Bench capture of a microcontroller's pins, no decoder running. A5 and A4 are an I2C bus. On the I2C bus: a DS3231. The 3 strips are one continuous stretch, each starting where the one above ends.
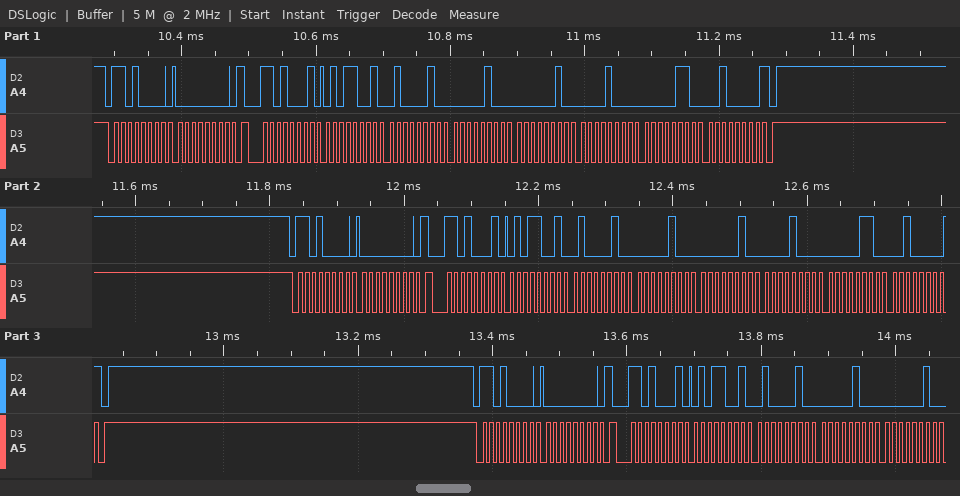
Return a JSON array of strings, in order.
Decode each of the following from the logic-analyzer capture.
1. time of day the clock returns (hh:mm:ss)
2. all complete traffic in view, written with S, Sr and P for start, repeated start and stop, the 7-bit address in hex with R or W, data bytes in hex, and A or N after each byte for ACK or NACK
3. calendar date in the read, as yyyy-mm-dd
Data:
["04:42:59", "S 68W A 00 A Sr 68R A 59 A 42 A 04 A 02 A 08 A 06 A 20 N P S 68W A 00 A Sr 68R A 59 A 42 A 04 A 02 A 08 A 06 A 20 N P S 68W A 00 A Sr 68R A 59 A 42 A 04 A 02 A", "2020-06-08"]
